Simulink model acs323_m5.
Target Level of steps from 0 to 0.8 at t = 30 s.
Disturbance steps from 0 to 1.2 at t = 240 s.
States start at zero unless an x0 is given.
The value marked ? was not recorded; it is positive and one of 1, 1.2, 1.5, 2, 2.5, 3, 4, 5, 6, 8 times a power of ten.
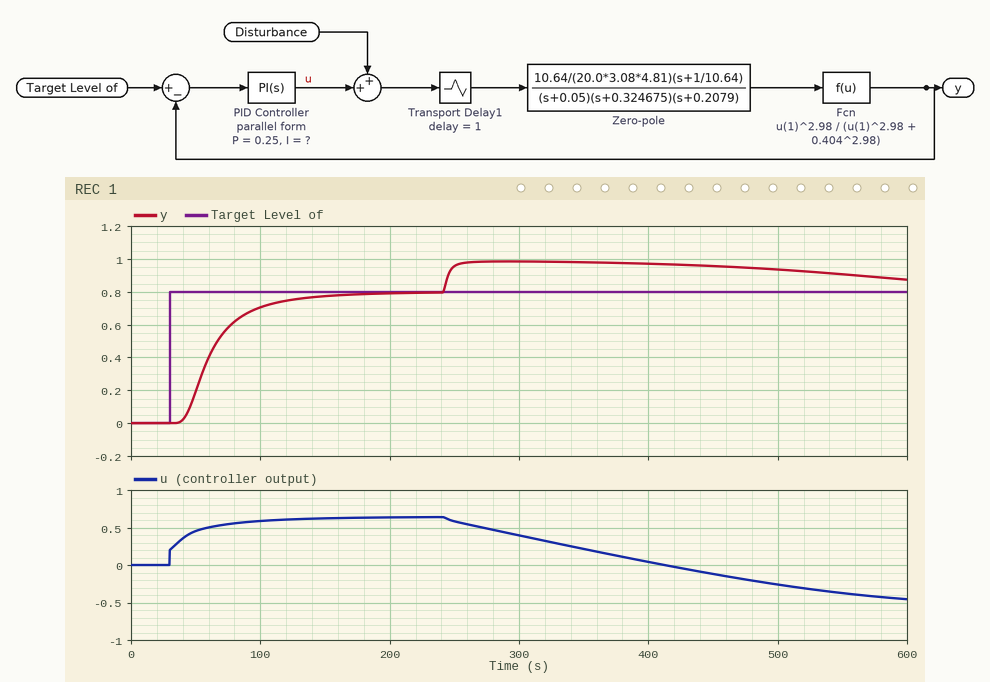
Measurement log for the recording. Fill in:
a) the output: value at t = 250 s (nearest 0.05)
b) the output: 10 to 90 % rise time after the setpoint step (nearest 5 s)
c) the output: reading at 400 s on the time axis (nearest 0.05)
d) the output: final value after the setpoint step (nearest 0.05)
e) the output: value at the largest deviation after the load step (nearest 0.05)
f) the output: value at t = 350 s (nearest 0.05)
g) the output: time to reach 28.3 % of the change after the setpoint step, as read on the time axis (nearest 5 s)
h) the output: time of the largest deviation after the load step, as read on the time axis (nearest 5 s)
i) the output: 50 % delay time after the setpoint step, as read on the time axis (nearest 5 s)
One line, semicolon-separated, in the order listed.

0.95; 60 s; 0.95; 0.80; 1.00; 1.00; 50 s; 290 s; 60 s
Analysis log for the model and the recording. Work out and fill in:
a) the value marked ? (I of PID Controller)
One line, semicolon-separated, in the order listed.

0.02
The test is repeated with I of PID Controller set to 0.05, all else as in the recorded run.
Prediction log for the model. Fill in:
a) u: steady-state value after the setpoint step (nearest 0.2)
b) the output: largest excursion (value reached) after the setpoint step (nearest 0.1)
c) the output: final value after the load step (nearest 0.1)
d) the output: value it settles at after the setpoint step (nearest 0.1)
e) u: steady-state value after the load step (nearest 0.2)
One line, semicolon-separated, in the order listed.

0.6; 0.8; 0.8; 0.8; -0.6
